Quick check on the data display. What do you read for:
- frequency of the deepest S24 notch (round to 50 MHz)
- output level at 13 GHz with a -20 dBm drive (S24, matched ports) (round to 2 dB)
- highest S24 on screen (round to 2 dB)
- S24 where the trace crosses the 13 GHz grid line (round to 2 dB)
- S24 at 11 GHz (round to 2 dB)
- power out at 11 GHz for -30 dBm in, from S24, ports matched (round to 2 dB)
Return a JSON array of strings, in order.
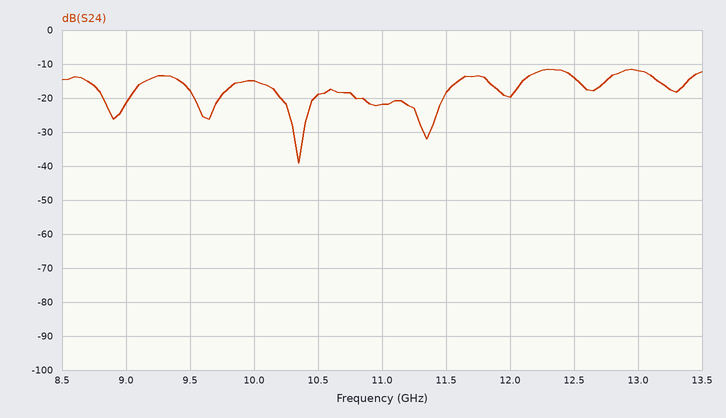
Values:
["10.35 GHz", "-32 dBm", "-12 dB", "-12 dB", "-22 dB", "-52 dBm"]
